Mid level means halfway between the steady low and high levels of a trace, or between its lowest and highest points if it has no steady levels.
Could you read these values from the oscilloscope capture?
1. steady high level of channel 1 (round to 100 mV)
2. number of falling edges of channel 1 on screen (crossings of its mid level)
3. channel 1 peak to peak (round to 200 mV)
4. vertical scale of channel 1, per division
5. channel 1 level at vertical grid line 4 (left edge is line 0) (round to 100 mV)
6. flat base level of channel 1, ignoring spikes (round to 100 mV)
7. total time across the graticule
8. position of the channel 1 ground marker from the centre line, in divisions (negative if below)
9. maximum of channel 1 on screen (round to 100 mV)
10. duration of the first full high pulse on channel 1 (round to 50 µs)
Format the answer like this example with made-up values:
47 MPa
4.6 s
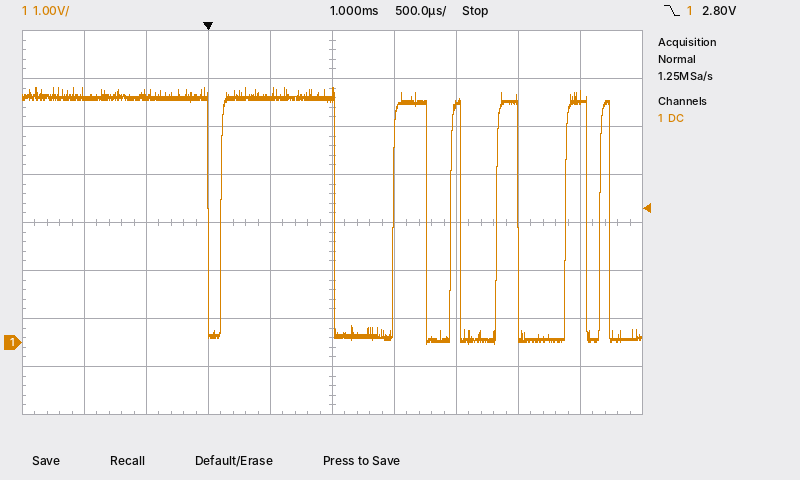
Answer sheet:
5.1 V
7
5.4 V
1 V
5.1 V
100 mV
5 ms
-2.5 div
5.3 V
900 µs
